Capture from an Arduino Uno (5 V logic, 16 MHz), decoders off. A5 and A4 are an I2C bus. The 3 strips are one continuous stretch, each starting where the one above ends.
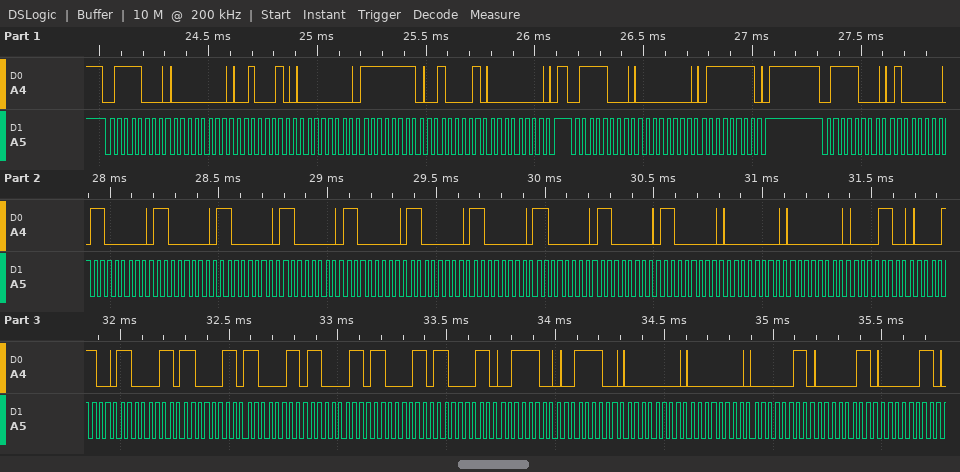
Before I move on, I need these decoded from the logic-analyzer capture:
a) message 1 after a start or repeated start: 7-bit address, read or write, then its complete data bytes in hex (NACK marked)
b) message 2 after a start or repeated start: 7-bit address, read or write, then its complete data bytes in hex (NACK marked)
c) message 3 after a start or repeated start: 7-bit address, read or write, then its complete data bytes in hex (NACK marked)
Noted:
0x3C write: 00 22 00 FF 21 00
0x3C write: 00 7F
0x3C write: 40 C0 C0 C0 C0 C0 C0 C0 C0 C0 C0 00 00 0C 0C C3 C3 C3 C3 C3 C3 3C 3C 00 00 03 03 03
